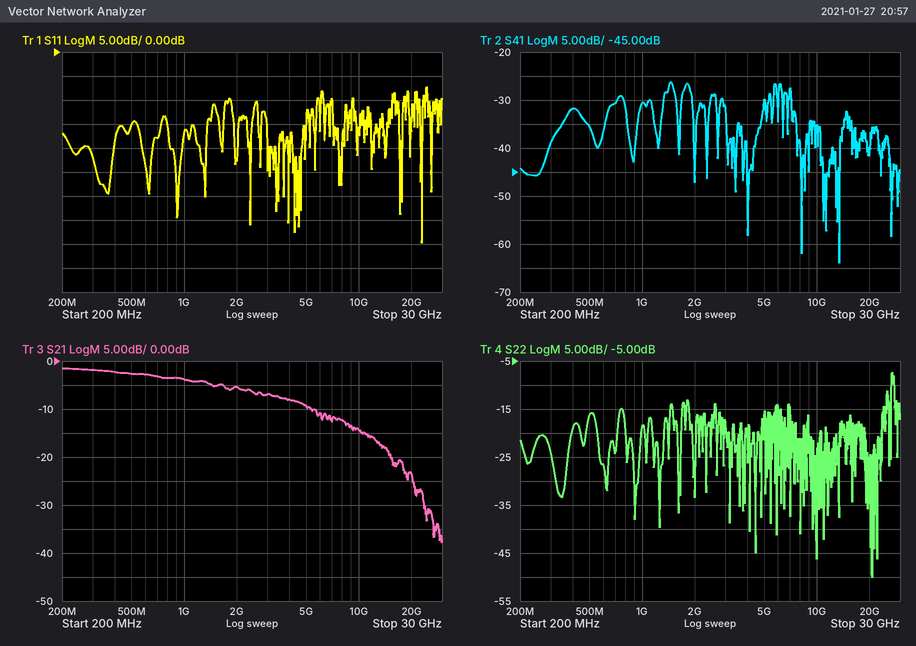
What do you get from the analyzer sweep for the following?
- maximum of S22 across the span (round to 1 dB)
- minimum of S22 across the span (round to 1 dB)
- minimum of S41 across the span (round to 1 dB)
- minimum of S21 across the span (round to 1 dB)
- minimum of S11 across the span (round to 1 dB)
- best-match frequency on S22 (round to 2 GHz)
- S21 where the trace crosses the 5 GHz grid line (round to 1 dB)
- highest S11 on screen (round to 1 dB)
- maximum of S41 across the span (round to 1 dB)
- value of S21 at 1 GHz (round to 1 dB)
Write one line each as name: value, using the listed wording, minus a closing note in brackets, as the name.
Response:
maximum of S22 across the span: -7 dB
minimum of S22 across the span: -50 dB
minimum of S41 across the span: -64 dB
minimum of S21 across the span: -38 dB
minimum of S11 across the span: -40 dB
best-match frequency on S22: 20 GHz
S21 where the trace crosses the 5 GHz grid line: -9 dB
highest S11 on screen: -7 dB
maximum of S41 across the span: -26 dB
value of S21 at 1 GHz: -4 dB
